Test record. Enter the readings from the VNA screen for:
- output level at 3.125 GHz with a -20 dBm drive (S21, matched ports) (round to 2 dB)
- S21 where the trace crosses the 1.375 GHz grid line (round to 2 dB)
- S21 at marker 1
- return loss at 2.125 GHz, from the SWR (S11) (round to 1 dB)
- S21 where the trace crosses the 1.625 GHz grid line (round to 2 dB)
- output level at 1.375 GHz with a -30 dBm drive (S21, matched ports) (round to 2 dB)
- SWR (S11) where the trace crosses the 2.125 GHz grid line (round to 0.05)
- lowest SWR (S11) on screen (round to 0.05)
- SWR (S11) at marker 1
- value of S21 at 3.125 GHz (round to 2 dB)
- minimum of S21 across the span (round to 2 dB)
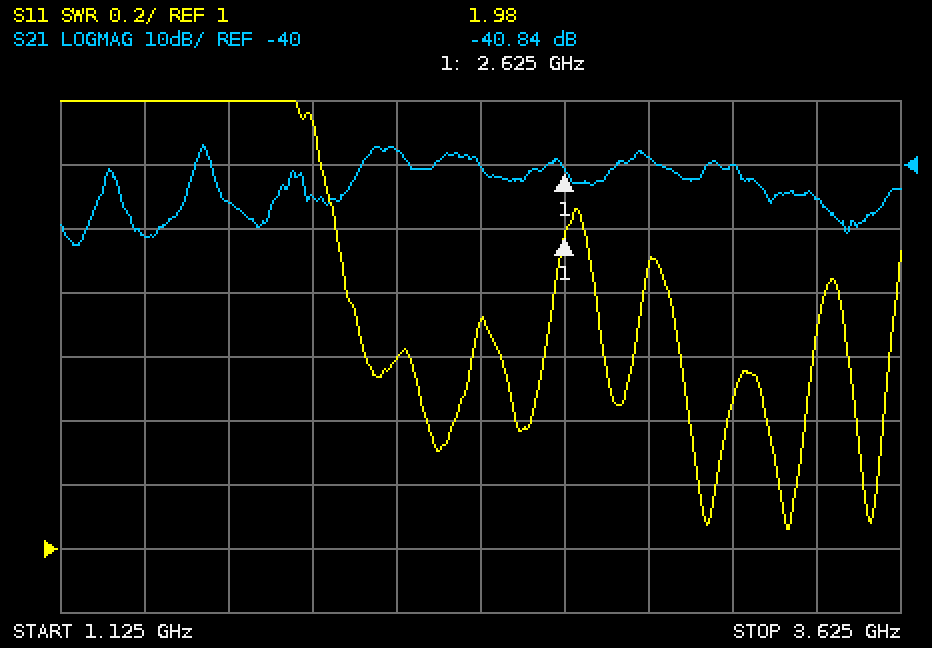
-60 dBm
-52 dB
-40.84 dB
13 dB
-46 dB
-82 dBm
1.60
1.05
1.98
-40 dB
-52 dB
